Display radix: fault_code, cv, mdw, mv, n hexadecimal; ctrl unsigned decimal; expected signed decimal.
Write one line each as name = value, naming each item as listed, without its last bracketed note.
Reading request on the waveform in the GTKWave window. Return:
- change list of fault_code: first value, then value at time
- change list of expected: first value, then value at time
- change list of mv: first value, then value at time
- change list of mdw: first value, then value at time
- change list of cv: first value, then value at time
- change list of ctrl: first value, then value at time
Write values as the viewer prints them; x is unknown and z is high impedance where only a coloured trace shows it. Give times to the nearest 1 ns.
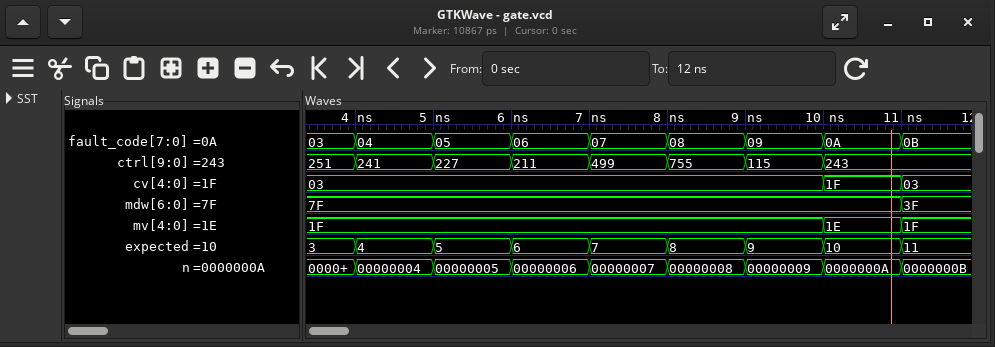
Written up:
change list of fault_code: first value, then value at time = 03, 04 at 4 ns, 05 at 5 ns, 06 at 6 ns, 07 at 7 ns, 08 at 8 ns, 09 at 9 ns, 0A at 10 ns, 0B at 11 ns
change list of expected: first value, then value at time = 3, 4 at 4 ns, 5 at 5 ns, 6 at 6 ns, 7 at 7 ns, 8 at 8 ns, 9 at 9 ns, 10 at 10 ns, 11 at 11 ns
change list of mv: first value, then value at time = 1F, 1E at 10 ns, 1F at 11 ns
change list of mdw: first value, then value at time = 7F, 3F at 11 ns
change list of cv: first value, then value at time = 03, 1F at 10 ns, 03 at 11 ns
change list of ctrl: first value, then value at time = 251, 241 at 4 ns, 227 at 5 ns, 211 at 6 ns, 499 at 7 ns, 755 at 8 ns, 115 at 9 ns, 243 at 10 ns
